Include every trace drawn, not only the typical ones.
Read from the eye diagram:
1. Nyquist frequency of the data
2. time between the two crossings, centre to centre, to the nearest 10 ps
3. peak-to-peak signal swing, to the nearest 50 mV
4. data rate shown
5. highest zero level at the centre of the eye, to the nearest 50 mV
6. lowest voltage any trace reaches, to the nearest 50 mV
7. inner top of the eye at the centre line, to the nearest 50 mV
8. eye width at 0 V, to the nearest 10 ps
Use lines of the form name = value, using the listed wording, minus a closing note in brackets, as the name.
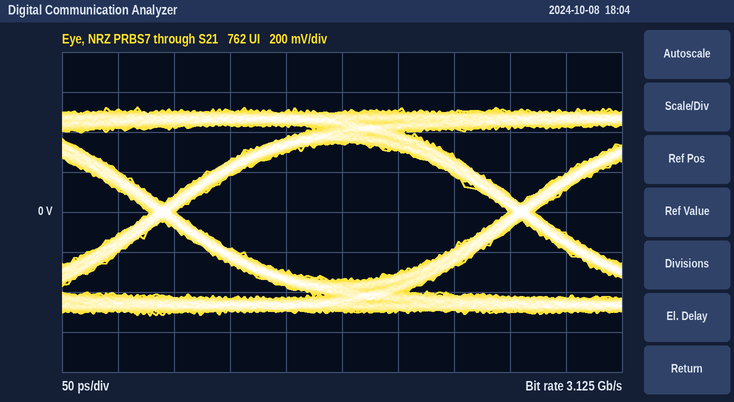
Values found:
Nyquist frequency of the data = 1.5625 GHz
time between the two crossings, centre to centre, to the nearest 10 ps = 320 ps
peak-to-peak signal swing, to the nearest 50 mV = 1.05 V
data rate shown = 3.125 Gb/s
highest zero level at the centre of the eye, to the nearest 50 mV = -350 mV
lowest voltage any trace reaches, to the nearest 50 mV = -500 mV
inner top of the eye at the centre line, to the nearest 50 mV = 350 mV
eye width at 0 V, to the nearest 10 ps = 300 ps
